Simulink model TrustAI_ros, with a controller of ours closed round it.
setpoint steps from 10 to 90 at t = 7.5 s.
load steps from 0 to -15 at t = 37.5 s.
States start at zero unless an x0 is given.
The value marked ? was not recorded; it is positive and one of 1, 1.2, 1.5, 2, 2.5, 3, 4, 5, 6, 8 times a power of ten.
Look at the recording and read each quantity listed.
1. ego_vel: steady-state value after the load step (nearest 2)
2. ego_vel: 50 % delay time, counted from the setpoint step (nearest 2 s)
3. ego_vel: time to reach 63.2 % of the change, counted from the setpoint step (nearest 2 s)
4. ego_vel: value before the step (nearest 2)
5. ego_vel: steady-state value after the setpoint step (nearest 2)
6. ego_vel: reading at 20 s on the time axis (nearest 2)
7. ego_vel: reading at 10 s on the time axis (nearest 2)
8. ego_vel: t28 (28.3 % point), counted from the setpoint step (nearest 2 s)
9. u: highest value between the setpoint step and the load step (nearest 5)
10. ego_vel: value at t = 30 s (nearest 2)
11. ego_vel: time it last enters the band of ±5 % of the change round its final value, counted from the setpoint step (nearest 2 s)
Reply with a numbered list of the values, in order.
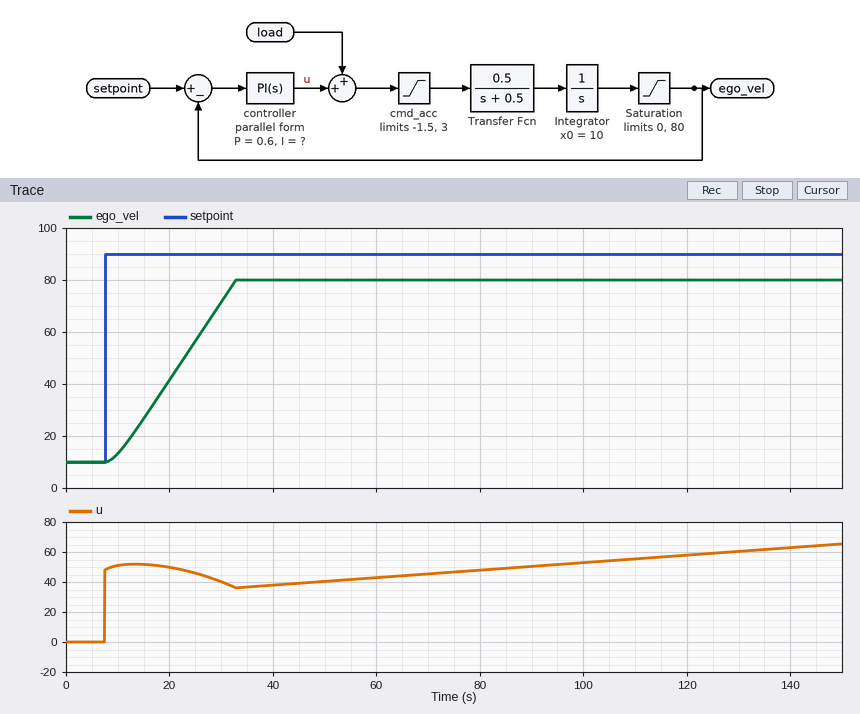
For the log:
1. 80
2. 14 s
3. 16 s
4. 10
5. 80
6. 42
7. 14
8. 8 s
9. 50
10. 72
11. 24 s
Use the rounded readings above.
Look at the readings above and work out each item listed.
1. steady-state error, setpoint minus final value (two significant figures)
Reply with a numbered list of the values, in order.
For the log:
1. 10
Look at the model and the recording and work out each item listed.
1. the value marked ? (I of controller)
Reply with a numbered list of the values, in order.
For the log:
1. 0.025
